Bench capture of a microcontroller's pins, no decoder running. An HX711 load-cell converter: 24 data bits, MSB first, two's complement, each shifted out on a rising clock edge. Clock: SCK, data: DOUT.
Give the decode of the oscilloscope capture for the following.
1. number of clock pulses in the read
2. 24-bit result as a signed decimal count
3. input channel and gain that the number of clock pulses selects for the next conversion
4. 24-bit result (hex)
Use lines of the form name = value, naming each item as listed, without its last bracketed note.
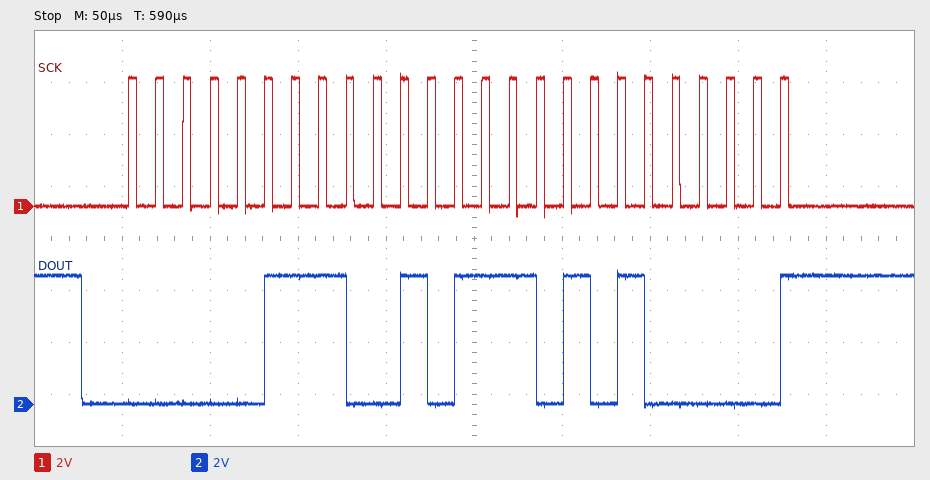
number of clock pulses in the read = 25
24-bit result as a signed decimal count = 470688
input channel and gain that the number of clock pulses selects for the next conversion = channel A, gain 128
24-bit result = 0x072EA0
